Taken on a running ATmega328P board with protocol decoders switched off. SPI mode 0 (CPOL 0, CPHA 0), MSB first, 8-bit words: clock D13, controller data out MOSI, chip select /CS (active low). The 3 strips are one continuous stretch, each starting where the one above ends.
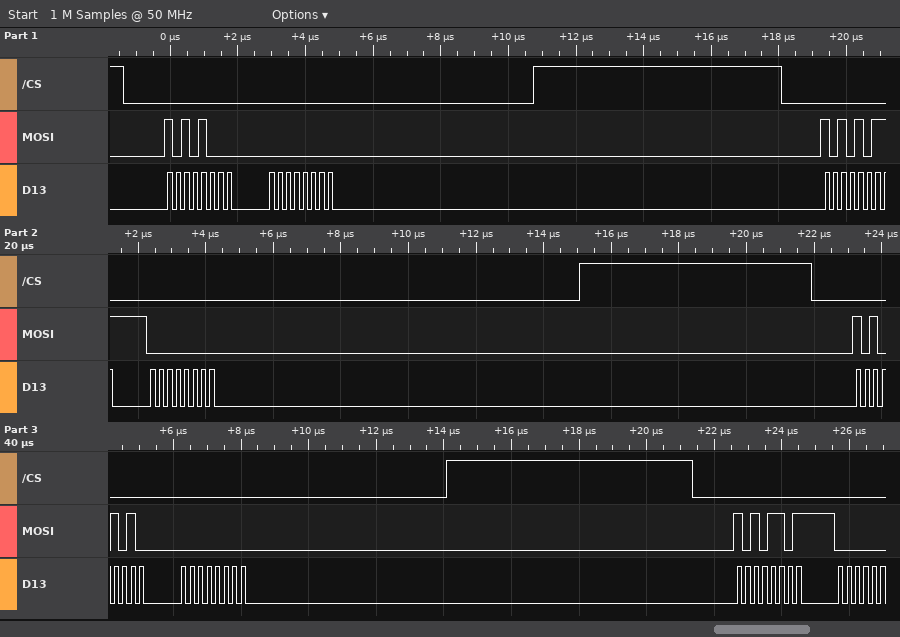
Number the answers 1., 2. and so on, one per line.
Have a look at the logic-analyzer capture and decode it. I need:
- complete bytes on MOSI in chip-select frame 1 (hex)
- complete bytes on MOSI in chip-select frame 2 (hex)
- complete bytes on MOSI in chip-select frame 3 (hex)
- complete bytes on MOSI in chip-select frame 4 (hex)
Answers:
1. A8 00
2. AB 00
3. AA 00
4. AD
